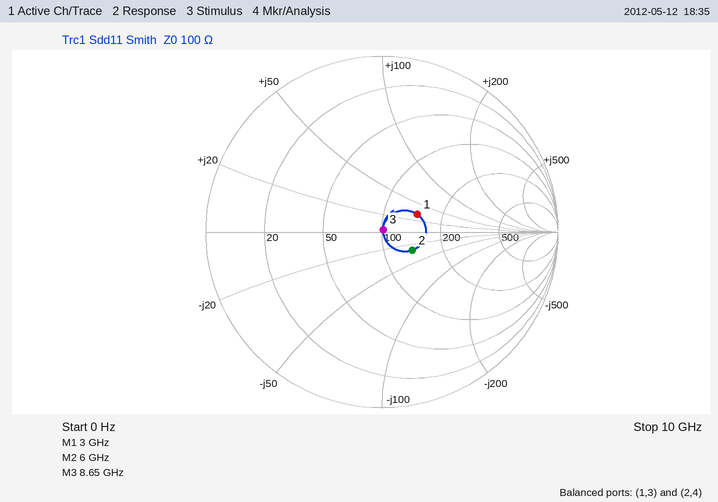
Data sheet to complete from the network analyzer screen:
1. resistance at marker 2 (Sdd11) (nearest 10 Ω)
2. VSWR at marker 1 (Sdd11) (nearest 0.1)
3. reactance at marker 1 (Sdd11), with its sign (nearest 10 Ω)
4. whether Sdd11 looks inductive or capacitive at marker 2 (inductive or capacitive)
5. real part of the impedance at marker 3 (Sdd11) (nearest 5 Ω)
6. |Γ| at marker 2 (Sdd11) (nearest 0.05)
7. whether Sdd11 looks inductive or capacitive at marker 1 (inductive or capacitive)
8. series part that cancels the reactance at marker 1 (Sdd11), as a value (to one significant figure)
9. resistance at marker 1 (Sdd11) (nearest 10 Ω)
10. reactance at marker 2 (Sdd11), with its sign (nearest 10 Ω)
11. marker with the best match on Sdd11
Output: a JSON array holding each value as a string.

["140 Ω", "1.6", "+30 Ω", "capacitive", "100 Ω", "0.20", "inductive", "2 pF", "150 Ω", "-30 Ω", "marker 3"]
